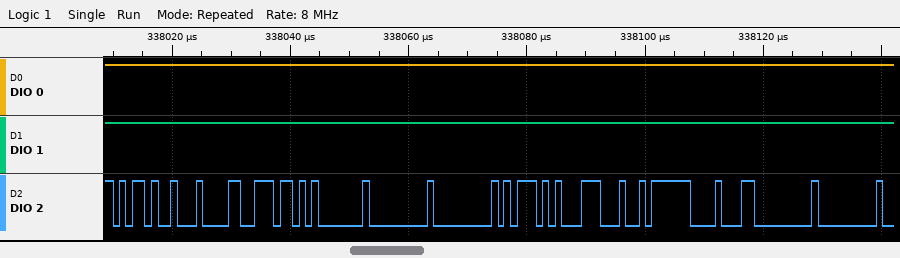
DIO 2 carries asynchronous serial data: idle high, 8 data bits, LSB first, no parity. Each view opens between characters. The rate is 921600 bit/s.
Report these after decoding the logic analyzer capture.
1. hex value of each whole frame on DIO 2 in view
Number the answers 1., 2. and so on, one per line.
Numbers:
1. 2D, 84, 6E, 01, 00, 00, 5D, 1C, FA, 88, 00, 00
